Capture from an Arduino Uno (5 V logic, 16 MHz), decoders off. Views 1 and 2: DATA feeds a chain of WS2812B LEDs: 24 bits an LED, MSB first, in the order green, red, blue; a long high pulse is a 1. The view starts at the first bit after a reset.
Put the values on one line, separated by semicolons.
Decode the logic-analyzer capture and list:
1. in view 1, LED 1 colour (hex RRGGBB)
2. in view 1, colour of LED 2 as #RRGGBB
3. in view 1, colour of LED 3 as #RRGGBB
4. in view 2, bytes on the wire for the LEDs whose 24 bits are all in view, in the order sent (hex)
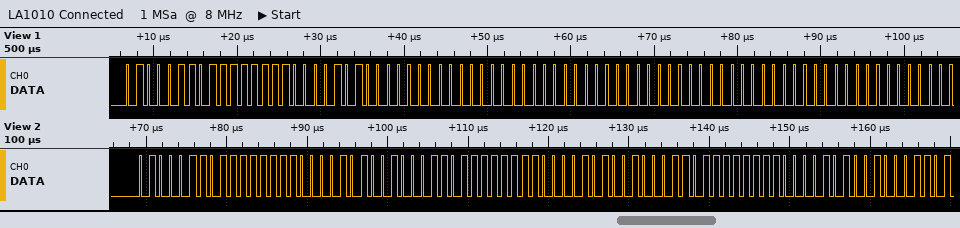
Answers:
#FF460A; #000000; #000000; 46 FF 0A 46 FF 0A 46 FF 0A
